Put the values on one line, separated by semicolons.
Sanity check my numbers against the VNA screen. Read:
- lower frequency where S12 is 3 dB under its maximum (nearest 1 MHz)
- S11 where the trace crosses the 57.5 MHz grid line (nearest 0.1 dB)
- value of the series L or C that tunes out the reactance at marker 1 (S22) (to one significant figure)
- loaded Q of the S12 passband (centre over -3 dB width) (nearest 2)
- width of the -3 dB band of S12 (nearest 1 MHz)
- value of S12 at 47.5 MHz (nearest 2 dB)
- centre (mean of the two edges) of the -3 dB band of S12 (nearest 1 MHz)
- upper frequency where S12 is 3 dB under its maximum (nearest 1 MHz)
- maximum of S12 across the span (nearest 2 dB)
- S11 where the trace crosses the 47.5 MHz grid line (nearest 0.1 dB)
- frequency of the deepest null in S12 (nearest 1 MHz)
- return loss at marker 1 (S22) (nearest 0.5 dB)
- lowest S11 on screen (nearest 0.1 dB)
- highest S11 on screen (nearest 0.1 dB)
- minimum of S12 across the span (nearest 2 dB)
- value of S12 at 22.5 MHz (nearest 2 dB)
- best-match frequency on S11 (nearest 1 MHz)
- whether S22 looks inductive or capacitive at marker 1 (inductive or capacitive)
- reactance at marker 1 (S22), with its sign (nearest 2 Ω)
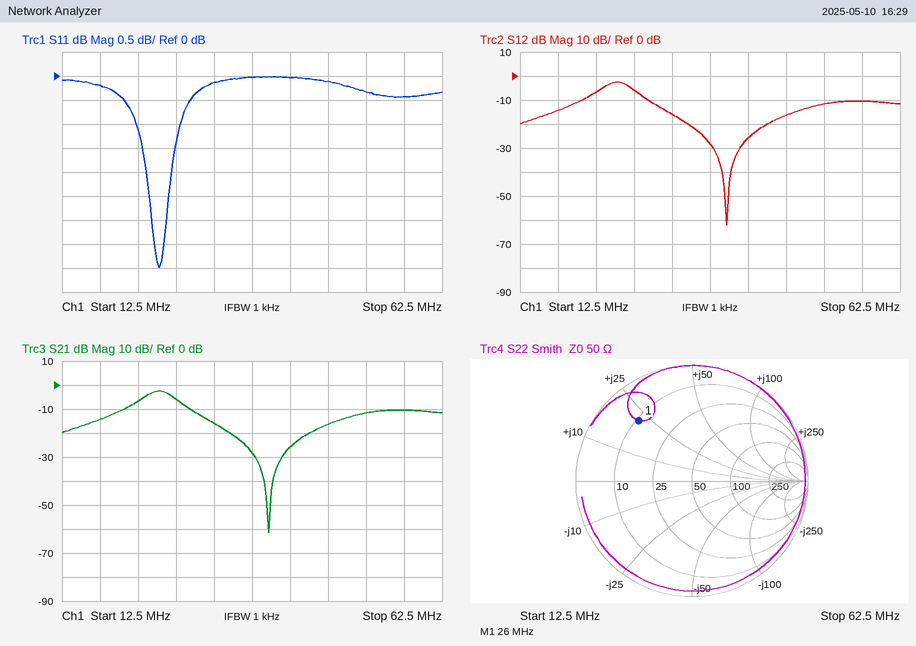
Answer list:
23 MHz; -0.4 dB; 300 pF; 6; 4 MHz; -16 dB; 25 MHz; 27 MHz; -2 dB; -0.1 dB; 40 MHz; 3.0 dB; -4.0 dB; 0.0 dB; -62 dB; -6 dB; 25 MHz; inductive; +22 Ω
